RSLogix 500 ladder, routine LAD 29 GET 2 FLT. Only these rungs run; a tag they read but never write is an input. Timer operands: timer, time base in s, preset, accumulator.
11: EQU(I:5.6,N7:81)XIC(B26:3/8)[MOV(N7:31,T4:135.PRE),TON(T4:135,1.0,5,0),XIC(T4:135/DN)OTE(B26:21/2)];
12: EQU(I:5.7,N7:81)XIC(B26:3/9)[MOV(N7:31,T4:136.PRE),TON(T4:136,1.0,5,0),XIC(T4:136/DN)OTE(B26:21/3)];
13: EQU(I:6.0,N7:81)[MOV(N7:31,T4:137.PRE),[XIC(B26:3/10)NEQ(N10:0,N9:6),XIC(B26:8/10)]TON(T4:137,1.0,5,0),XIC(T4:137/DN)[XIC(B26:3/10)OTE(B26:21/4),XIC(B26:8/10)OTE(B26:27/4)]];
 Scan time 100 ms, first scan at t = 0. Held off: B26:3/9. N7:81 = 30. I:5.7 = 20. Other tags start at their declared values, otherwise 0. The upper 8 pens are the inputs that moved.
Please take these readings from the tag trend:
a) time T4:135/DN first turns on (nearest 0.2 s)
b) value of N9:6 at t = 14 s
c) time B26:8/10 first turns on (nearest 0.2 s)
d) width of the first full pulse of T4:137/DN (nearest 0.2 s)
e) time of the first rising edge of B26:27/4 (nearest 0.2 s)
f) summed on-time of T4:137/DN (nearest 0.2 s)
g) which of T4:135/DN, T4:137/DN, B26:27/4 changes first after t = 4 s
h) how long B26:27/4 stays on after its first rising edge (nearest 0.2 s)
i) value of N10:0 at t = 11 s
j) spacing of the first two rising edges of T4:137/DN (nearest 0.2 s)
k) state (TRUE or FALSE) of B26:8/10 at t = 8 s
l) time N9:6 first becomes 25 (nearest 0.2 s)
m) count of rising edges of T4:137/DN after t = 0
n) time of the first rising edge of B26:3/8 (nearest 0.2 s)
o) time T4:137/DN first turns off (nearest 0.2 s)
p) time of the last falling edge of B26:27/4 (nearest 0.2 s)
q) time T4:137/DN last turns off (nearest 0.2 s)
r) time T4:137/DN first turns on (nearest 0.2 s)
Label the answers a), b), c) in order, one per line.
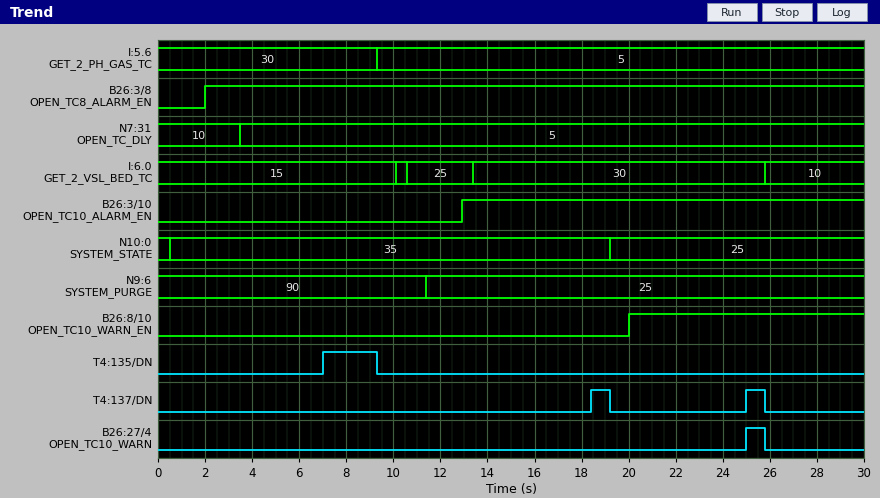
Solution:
a) 7.0 s
b) 25
c) 20.0 s
d) 0.8 s
e) 25.0 s
f) 1.6 s
g) T4:135/DN
h) 0.8 s
i) 35
j) 6.6 s
k) FALSE
l) 11.4 s
m) 2
n) 2.0 s
o) 19.2 s
p) 25.8 s
q) 25.8 s
r) 18.4 s
